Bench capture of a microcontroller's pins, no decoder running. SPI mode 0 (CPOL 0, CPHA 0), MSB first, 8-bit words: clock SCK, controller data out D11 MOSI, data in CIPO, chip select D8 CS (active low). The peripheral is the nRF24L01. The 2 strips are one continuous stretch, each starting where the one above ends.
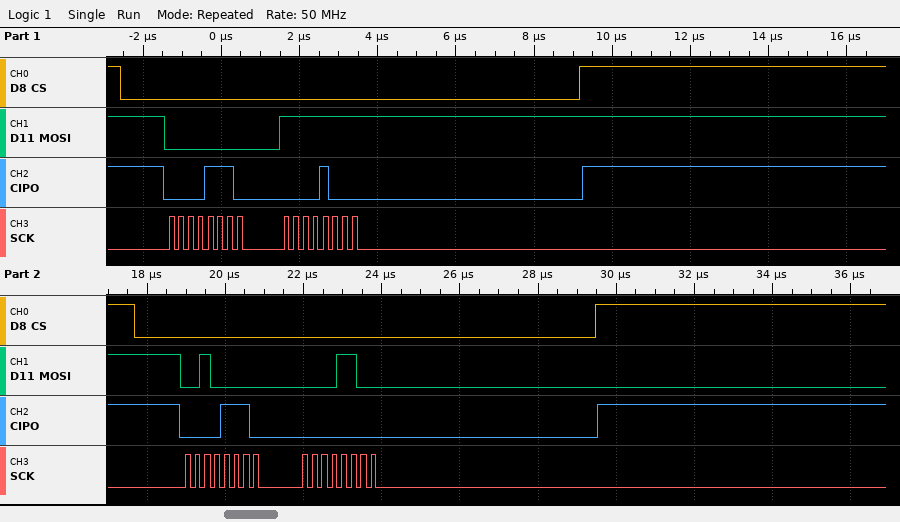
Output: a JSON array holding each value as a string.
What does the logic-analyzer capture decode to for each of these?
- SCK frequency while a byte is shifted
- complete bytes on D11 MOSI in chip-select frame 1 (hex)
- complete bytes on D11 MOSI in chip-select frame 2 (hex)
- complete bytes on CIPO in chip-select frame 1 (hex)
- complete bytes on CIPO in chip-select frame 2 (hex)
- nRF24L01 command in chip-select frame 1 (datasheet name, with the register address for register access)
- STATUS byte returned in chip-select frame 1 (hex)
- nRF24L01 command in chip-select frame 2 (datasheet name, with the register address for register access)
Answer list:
["4 MHz", "00 FF", "20 0C", "0E 08", "0E 00", "R_REGISTER 0x00", "0x0E", "W_REGISTER 0x00"]
